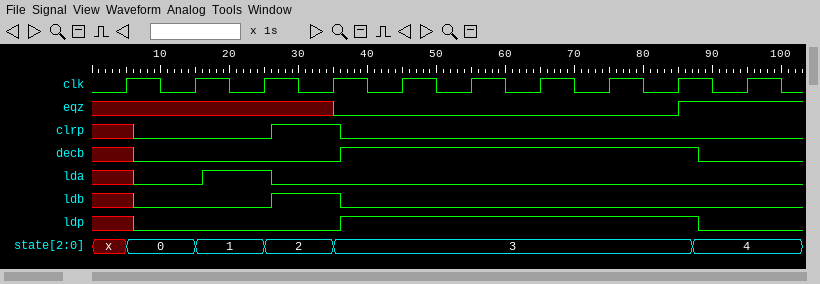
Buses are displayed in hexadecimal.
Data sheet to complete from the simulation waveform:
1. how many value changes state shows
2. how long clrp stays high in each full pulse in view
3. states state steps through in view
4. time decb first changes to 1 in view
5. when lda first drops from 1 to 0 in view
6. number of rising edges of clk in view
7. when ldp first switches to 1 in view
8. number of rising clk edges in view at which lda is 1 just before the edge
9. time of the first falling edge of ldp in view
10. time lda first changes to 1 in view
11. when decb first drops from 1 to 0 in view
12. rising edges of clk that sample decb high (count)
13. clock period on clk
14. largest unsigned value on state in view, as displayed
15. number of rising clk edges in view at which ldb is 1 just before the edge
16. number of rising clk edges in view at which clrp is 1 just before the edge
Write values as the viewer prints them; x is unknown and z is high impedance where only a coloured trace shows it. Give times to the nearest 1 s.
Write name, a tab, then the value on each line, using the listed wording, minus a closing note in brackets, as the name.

how many value changes state shows	5
how long clrp stays high in each full pulse in view	10 s
states state steps through in view	x, 0, 1, 2, 3, 4
time decb first changes to 1 in view	36 s
when lda first drops from 1 to 0 in view	26 s
number of rising edges of clk in view	10
when ldp first switches to 1 in view	36 s
number of rising clk edges in view at which lda is 1 just before the edge	1
time of the first falling edge of ldp in view	88 s
time lda first changes to 1 in view	16 s
when decb first drops from 1 to 0 in view	88 s
rising edges of clk that sample decb high	5
clock period on clk	10 s
largest unsigned value on state in view, as displayed	4
number of rising clk edges in view at which ldb is 1 just before the edge	1
number of rising clk edges in view at which clrp is 1 just before the edge	1
